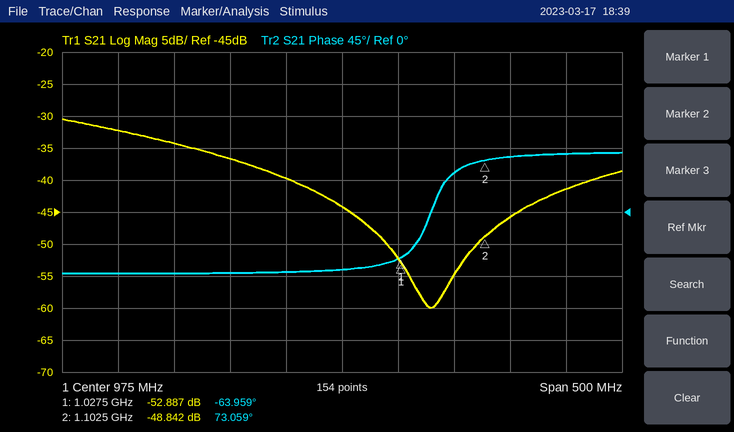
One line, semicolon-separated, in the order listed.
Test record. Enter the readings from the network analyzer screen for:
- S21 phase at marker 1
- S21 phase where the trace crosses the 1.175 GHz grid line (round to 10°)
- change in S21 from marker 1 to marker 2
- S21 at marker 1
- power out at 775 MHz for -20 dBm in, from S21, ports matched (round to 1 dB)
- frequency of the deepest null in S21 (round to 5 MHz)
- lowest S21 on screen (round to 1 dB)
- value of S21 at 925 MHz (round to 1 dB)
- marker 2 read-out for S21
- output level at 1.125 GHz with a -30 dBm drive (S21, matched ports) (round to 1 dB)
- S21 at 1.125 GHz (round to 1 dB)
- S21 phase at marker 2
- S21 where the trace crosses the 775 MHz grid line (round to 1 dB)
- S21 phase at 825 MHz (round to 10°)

-63.959°; 80°; 4.045 dB; -52.887 dB; -52 dBm; 1.055 GHz; -60 dB; -40 dB; -48.842 dB; -76 dBm; -46 dB; 73.059°; -32 dB; -90°
